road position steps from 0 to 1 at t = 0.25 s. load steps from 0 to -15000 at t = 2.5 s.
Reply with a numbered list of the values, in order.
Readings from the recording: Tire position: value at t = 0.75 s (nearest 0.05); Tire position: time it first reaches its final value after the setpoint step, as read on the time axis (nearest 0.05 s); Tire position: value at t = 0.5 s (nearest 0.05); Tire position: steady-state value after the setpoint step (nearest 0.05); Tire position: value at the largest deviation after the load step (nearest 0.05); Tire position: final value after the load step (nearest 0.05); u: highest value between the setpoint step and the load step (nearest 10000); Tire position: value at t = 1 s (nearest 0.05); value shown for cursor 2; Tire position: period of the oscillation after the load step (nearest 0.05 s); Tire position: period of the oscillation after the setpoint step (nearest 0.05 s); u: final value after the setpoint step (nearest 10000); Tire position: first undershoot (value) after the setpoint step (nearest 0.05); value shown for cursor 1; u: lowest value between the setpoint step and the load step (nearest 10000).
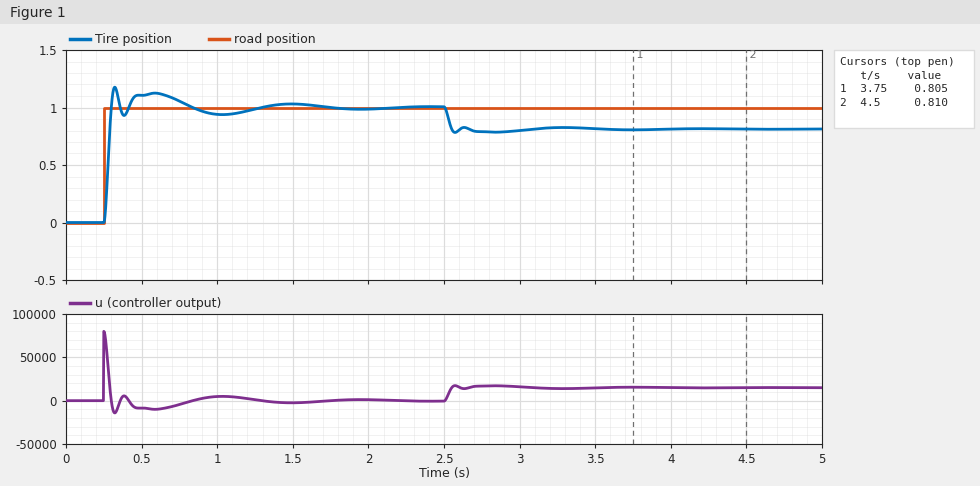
1. 1.05
2. 0.30 s
3. 1.10
4. 1.00
5. 0.80
6. 0.80
7. 80000
8. 0.95
9. 0.810
10. 0.25 s
11. 0.25 s
12. 0
13. 0.95
14. 0.805
15. -10000
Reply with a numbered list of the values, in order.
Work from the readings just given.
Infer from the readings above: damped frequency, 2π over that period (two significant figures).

1. 25 rad/s
